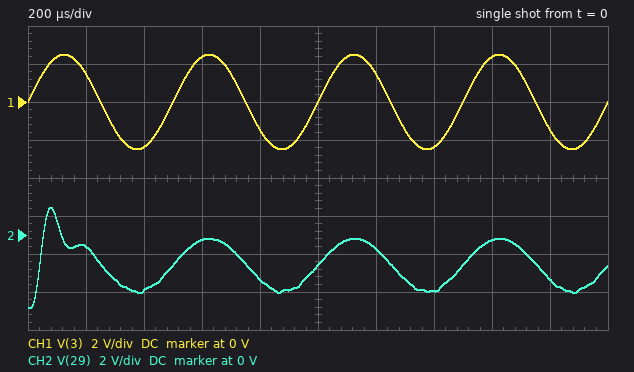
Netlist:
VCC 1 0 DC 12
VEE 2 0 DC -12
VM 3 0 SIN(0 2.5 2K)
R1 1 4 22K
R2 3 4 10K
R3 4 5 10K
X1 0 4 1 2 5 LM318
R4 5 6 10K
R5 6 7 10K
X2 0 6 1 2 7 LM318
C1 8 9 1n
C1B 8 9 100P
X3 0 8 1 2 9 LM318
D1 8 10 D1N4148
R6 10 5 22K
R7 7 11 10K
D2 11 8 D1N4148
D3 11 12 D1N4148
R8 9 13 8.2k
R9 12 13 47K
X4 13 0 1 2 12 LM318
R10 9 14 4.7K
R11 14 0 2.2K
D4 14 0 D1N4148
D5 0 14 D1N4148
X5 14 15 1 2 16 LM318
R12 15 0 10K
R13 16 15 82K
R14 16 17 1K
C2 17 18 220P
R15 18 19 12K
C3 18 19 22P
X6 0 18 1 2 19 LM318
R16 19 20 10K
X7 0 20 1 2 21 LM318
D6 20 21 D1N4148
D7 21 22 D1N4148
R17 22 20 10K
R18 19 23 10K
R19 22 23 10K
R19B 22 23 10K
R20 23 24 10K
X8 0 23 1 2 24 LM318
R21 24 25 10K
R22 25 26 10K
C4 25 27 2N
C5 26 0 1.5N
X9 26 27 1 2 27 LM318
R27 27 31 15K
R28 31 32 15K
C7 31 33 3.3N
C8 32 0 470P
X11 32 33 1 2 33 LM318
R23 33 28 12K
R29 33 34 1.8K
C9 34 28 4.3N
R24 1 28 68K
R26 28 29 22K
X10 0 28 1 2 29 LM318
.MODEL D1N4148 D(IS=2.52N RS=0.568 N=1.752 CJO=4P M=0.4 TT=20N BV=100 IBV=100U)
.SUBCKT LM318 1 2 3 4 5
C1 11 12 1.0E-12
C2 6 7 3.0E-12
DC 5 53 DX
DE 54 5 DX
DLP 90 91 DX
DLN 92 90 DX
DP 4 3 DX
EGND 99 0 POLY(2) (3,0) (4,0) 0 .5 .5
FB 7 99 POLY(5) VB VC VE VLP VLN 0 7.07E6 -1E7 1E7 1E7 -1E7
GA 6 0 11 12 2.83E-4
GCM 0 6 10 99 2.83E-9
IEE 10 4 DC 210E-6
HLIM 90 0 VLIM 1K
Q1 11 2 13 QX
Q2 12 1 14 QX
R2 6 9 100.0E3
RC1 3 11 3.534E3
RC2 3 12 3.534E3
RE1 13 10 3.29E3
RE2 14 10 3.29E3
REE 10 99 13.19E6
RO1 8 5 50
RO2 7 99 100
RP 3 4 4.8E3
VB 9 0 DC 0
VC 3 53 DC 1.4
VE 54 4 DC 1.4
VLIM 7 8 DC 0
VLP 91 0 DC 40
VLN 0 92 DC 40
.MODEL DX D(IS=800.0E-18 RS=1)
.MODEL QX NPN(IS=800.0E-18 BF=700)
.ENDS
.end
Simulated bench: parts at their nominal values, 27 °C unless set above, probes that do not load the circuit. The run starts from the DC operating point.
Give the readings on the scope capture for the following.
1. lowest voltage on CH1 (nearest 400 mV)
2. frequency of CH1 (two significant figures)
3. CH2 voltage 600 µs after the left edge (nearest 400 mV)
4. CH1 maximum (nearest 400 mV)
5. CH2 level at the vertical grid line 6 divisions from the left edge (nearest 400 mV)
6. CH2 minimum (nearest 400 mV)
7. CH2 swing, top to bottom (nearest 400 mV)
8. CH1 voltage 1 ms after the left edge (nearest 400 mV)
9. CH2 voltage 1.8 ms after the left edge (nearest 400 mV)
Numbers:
-2.4 V
2.0 kHz
-400 mV
2.4 V
-800 mV
-4.0 V
5.2 V
0 V
-2.4 V
